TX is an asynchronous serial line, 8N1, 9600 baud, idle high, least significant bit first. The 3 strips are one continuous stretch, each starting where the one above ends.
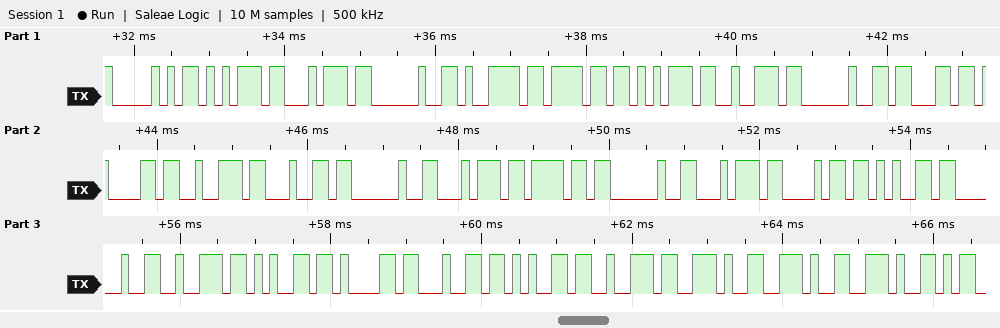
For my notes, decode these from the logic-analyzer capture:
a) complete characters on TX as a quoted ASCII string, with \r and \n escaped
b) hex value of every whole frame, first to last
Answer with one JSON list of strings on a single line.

["\"Put your card to the reader...\"", "50 75 74 20 79 6F 75 72 20 63 61 72 64 20 74 6F 20 74 68 65 20 72 65 61 64 65 72 2E 2E 2E"]
